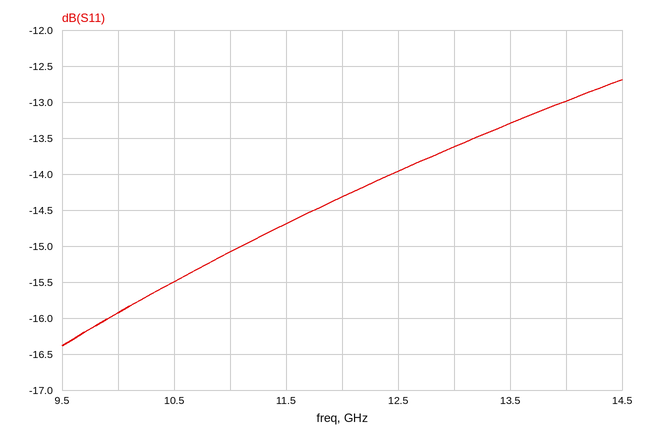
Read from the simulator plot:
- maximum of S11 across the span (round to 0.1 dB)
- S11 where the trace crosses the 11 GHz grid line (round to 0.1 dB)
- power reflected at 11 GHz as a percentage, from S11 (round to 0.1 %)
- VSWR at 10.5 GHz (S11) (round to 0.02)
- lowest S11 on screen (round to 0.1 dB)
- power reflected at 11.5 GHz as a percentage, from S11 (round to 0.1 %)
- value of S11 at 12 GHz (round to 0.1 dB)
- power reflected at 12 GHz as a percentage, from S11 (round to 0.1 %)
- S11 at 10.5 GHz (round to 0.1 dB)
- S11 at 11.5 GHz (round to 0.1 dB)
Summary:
-12.7 dB
-15.1 dB
3.1 %
1.40
-16.4 dB
3.4 %
-14.3 dB
3.7 %
-15.5 dB
-14.7 dB
